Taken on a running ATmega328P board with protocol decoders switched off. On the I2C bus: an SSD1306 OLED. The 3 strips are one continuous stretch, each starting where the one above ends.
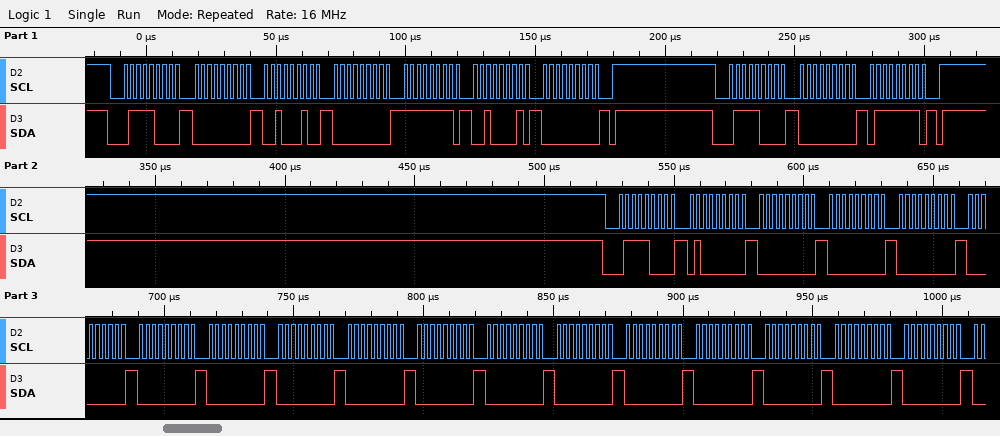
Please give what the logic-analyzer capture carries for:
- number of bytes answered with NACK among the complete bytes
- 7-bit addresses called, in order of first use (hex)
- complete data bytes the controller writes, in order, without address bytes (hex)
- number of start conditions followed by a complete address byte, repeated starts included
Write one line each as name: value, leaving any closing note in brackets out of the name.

number of bytes answered with NACK among the complete bytes: 0
7-bit addresses called, in order of first use: 0x3C
complete data bytes the controller writes, in order, without address bytes: 00 22 00 FF 21 00 00 7F 40 00 00 00 00 00 00 00 00 00 00 00 00 00 00 00 00
number of start conditions followed by a complete address byte, repeated starts included: 3
